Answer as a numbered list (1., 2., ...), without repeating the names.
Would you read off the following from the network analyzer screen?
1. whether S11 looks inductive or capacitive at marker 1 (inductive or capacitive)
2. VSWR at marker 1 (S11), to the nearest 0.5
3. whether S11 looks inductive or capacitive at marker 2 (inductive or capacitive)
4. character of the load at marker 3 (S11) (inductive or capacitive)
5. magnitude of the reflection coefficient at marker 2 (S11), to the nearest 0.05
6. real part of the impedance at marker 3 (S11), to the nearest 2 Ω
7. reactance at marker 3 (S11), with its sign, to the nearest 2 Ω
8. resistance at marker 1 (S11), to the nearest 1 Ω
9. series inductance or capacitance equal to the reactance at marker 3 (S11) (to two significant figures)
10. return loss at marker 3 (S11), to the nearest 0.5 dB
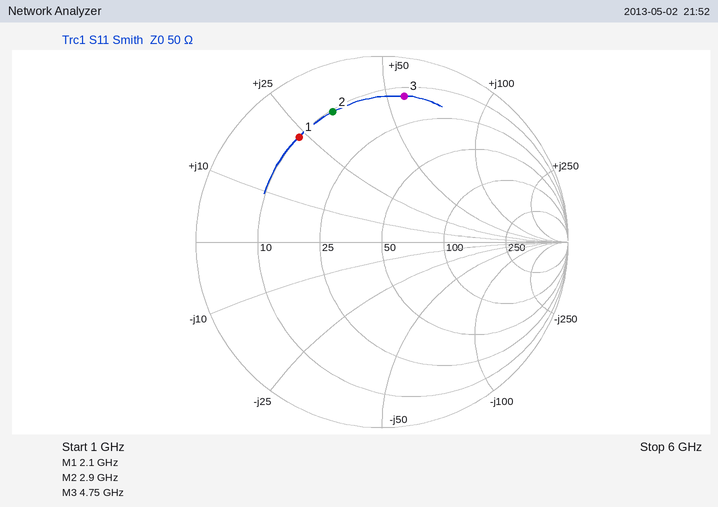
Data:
1. inductive
2. 6.0
3. inductive
4. inductive
5. 0.75
6. 14 Ω
7. +56 Ω
8. 10 Ω
9. 1.9 nH
10. 2.0 dB
